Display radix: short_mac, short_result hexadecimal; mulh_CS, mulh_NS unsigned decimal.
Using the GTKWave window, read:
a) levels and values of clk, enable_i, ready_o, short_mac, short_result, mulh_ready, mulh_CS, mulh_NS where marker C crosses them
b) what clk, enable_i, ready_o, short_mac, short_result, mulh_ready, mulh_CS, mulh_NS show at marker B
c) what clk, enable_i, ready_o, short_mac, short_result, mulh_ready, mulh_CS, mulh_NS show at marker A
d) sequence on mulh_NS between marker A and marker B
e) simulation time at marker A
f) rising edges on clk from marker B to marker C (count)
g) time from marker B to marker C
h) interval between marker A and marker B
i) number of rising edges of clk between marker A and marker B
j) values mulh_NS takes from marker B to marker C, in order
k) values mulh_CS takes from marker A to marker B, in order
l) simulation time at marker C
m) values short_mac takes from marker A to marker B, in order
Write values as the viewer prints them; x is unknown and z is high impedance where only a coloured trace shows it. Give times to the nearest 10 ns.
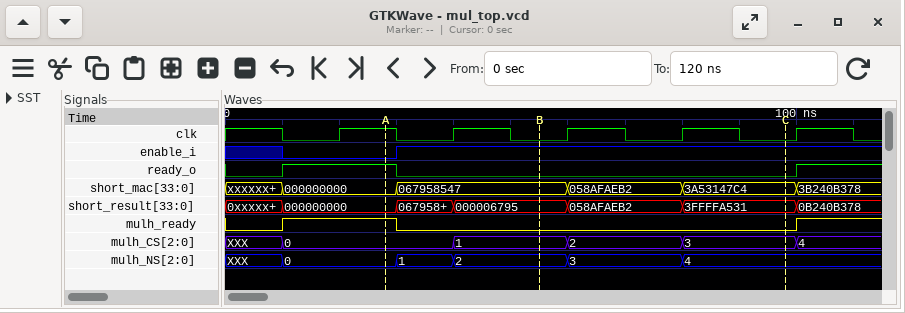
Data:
clk=0, enable_i=1, ready_o=0, short_mac=3A53147C4, short_result=3FFFFA531, mulh_ready=0, mulh_CS=3, mulh_NS=4
clk=0, enable_i=1, ready_o=0, short_mac=067958547, short_result=000006795, mulh_ready=0, mulh_CS=1, mulh_NS=2
clk=1, enable_i=0, ready_o=1, short_mac=000000000, short_result=000000000, mulh_ready=1, mulh_CS=0, mulh_NS=0
0, 1, 2
30 ns
2
40 ns
30 ns
1
2, 3, 4
0, 1
100 ns
000000000, 067958547
